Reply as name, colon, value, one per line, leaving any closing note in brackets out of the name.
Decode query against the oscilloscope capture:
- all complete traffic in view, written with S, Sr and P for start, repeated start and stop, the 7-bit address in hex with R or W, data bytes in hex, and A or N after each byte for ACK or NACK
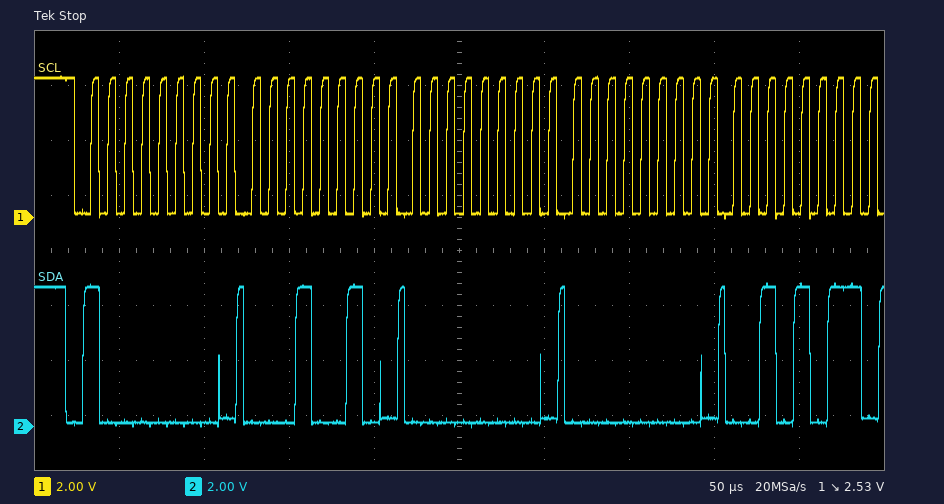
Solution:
all complete traffic in view, written with S, Sr and P for start, repeated start and stop, the 7-bit address in hex with R or W, data bytes in hex, and A or N after each byte for ACK or NACK: S 40W A 12 A 00 A 00 A 2B A
